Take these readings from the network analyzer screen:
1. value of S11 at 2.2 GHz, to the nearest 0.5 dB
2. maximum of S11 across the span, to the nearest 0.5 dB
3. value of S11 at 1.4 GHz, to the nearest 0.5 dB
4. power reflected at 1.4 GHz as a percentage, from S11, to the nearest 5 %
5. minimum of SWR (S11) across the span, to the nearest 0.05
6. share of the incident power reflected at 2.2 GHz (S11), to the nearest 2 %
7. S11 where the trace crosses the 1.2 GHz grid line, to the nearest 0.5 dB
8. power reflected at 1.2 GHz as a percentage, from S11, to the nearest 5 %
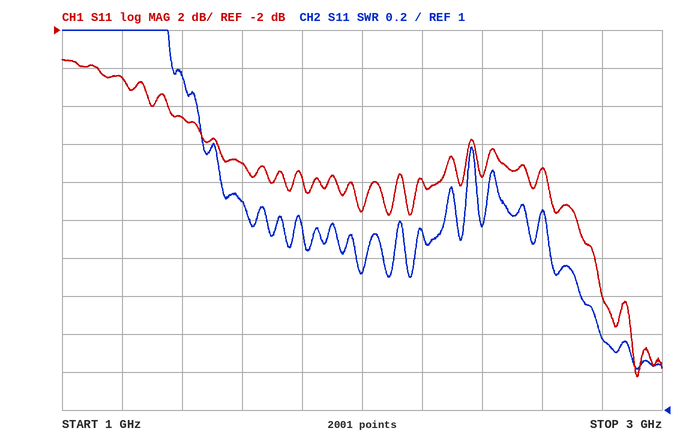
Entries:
-10.0 dB
-3.5 dB
-6.5 dB
20 %
1.20
10 %
-4.5 dB
35 %
